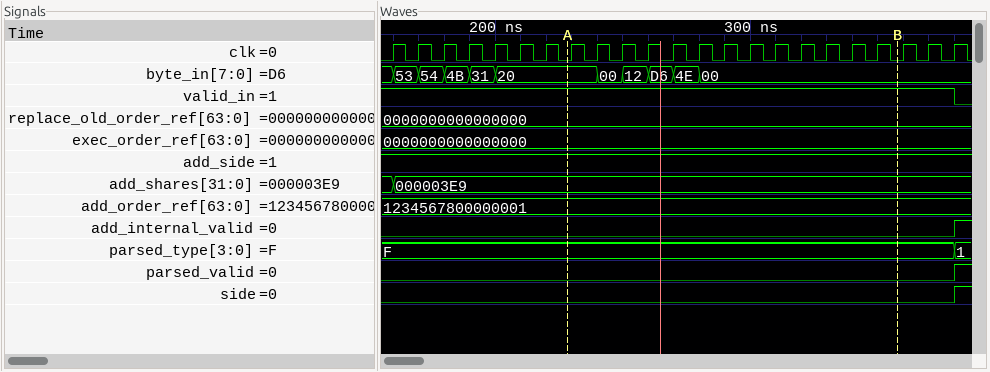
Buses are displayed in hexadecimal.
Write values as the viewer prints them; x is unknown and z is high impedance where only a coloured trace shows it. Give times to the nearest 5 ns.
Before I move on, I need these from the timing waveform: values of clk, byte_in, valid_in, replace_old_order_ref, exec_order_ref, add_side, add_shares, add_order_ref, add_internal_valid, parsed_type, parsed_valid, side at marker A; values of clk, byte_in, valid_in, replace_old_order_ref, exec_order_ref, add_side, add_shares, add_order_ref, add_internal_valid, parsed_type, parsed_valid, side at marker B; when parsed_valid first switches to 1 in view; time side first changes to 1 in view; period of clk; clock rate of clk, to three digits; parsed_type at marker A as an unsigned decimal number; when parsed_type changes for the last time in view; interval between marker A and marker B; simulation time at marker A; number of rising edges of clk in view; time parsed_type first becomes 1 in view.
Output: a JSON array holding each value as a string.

["clk=0, byte_in=20, valid_in=1, replace_old_order_ref=0000000000000000, exec_order_ref=0000000000000000, add_side=1, add_shares=000003E9, add_order_ref=1234567800000001, add_internal_valid=0, parsed_type=F, parsed_valid=0, side=0", "clk=0, byte_in=00, valid_in=1, replace_old_order_ref=0000000000000000, exec_order_ref=0000000000000000, add_side=1, add_shares=000003E9, add_order_ref=1234567800000001, add_internal_valid=0, parsed_type=F, parsed_valid=0, side=0", "380 ns", "380 ns", "10 ns", "100 MHz", "15", "380 ns", "130 ns", "230 ns", "23", "380 ns"]
